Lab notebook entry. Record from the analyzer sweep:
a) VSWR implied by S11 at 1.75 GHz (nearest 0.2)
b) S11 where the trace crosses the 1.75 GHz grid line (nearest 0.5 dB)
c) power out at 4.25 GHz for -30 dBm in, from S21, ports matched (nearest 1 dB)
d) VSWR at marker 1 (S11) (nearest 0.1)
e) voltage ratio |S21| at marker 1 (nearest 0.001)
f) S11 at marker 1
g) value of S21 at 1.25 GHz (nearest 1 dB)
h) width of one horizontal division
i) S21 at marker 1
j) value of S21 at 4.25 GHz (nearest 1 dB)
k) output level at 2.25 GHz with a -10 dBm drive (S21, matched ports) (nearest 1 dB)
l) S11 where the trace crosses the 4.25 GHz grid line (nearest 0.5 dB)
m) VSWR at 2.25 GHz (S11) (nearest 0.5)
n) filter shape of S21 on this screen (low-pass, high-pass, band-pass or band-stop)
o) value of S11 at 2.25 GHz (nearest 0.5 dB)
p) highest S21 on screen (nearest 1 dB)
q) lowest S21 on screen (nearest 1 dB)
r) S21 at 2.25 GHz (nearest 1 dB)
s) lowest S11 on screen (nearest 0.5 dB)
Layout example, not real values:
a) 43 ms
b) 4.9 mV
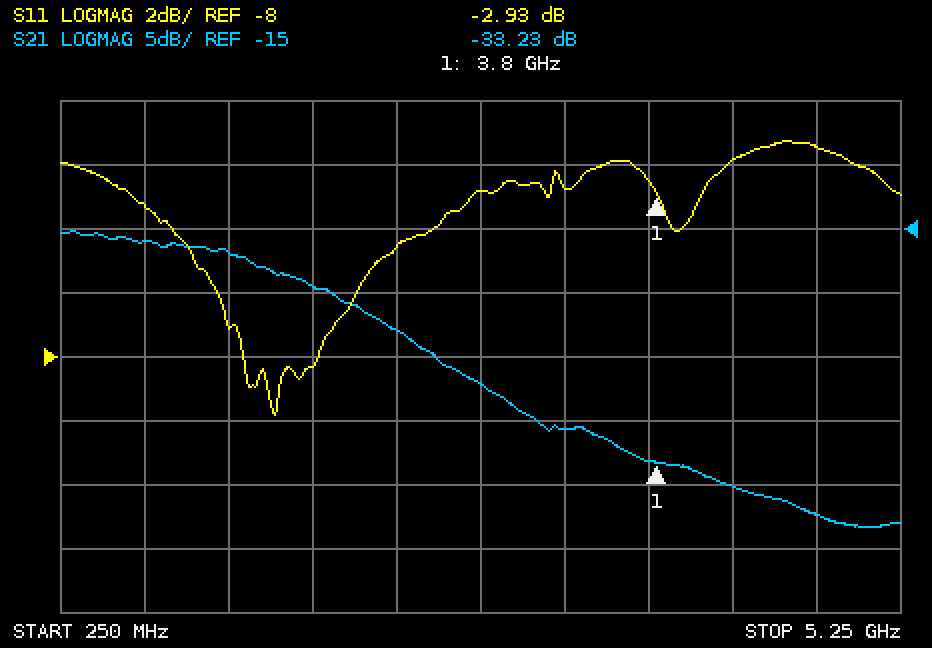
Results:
a) 2.2
b) -8.5 dB
c) -65 dBm
d) 6.0
e) 0.022
f) -2.93 dB
g) -17 dB
h) 500 MHz
i) -33.23 dB
j) -35 dB
k) -33 dBm
l) -2.0 dB
m) 4.0
n) low-pass
o) -4.5 dB
p) -15 dB
q) -38 dB
r) -23 dB
s) -10.0 dB
